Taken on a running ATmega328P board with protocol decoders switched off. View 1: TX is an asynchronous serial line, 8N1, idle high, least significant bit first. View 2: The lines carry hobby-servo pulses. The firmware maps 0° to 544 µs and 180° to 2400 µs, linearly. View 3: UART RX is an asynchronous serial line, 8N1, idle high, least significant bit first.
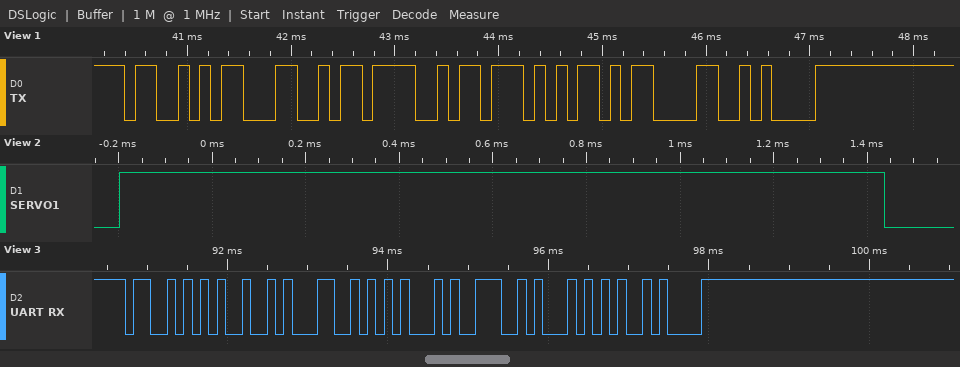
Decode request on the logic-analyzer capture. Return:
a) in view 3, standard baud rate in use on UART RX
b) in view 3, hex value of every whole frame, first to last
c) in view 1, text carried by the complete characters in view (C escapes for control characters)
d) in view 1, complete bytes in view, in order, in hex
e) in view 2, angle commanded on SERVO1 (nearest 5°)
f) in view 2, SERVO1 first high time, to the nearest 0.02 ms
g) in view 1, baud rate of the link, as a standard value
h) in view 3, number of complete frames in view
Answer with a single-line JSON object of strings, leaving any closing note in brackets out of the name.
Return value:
{"in view 3, standard baud rate in use on UART RX": "9600 baud", "in view 3, hex value of every whole frame, first to last": "53 49 4C 45 4E 54 0A", "in view 1, text carried by the complete characters in view": "\"SLOW\\r\\n\"", "in view 1, complete bytes in view, in order, in hex": "53 4C 4F 57 0D 0A", "in view 2, angle commanded on SERVO1": "105°", "in view 2, SERVO1 first high time, to the nearest 0.02 ms": "1.64 ms", "in view 1, baud rate of the link, as a standard value": "9600 baud", "in view 3, number of complete frames in view": "7"}
